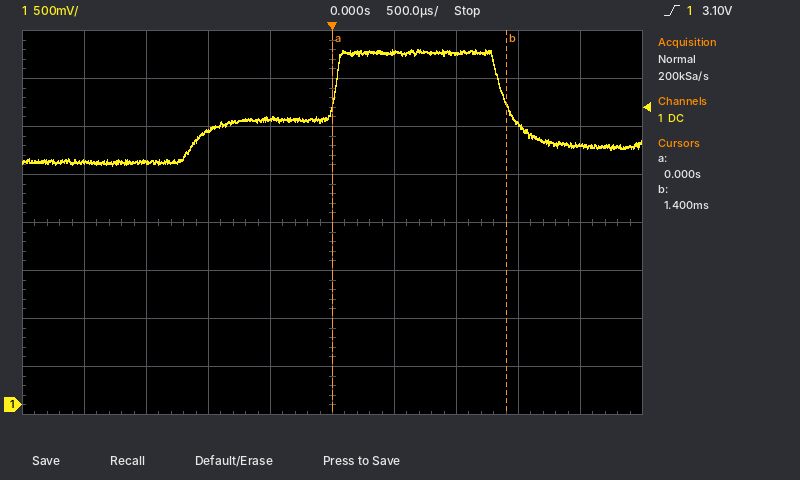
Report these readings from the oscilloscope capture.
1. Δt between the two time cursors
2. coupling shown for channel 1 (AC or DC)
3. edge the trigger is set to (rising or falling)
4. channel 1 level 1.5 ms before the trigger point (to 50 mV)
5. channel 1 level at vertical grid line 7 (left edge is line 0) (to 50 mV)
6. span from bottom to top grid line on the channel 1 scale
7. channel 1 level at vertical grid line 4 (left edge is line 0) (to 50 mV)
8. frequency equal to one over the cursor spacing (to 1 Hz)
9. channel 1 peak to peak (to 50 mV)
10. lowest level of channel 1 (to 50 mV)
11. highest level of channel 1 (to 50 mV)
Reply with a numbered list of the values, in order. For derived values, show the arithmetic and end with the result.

1. 1.4 ms − (0 s) = 1.40 ms
2. DC
3. rising
4. 2.55 V
5. 3.65 V
6. 4 V
7. 3.00 V
8. 1 / 1.40 ms ≈ 714 Hz
9. 3.70 V − (2.50 V) = 1.20 V
10. 2.50 V
11. 3.70 V
